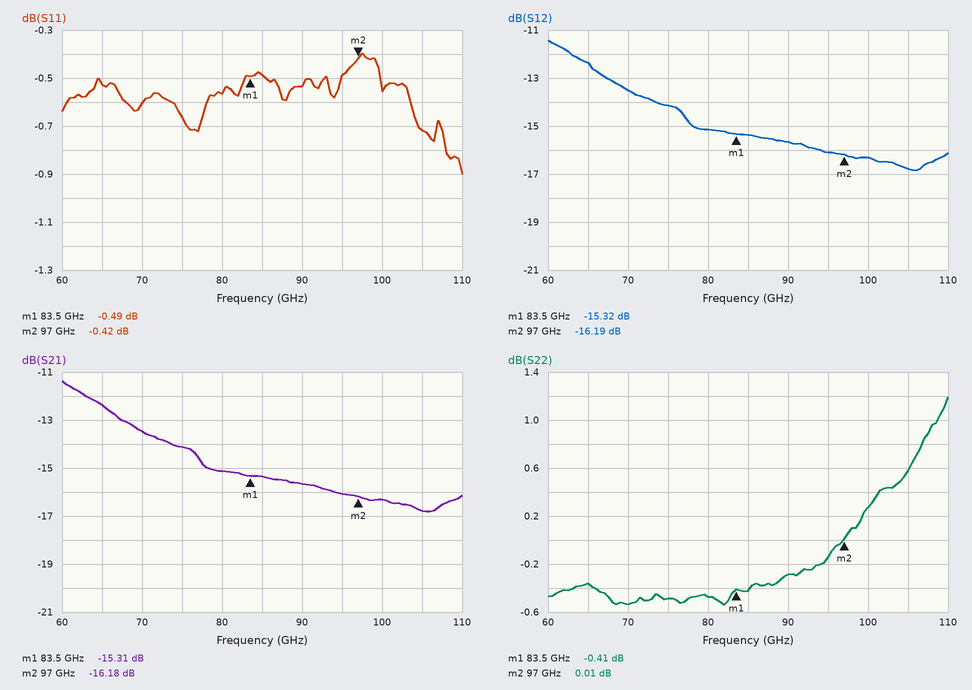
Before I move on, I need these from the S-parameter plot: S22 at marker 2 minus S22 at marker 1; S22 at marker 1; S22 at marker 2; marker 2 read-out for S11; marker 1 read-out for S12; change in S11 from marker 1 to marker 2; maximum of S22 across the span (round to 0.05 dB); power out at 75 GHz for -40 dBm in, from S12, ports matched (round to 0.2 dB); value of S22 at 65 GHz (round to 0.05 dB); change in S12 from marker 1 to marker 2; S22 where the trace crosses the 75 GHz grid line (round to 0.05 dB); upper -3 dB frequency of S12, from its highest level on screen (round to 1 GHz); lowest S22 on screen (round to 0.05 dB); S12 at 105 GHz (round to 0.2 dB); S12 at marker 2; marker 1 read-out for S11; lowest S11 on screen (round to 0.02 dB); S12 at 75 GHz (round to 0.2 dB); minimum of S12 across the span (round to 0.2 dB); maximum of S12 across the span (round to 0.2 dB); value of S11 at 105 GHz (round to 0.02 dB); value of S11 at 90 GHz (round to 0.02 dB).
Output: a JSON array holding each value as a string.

["0.42 dB", "-0.41 dB", "0.01 dB", "-0.42 dB", "-15.32 dB", "0.07 dB", "1.20 dB", "-54.2 dBm", "-0.35 dB", "-0.87 dB", "-0.50 dB", "77 GHz", "-0.55 dB", "-16.8 dB", "-16.19 dB", "-0.49 dB", "-0.90 dB", "-14.2 dB", "-16.8 dB", "-11.4 dB", "-0.72 dB", "-0.54 dB"]
